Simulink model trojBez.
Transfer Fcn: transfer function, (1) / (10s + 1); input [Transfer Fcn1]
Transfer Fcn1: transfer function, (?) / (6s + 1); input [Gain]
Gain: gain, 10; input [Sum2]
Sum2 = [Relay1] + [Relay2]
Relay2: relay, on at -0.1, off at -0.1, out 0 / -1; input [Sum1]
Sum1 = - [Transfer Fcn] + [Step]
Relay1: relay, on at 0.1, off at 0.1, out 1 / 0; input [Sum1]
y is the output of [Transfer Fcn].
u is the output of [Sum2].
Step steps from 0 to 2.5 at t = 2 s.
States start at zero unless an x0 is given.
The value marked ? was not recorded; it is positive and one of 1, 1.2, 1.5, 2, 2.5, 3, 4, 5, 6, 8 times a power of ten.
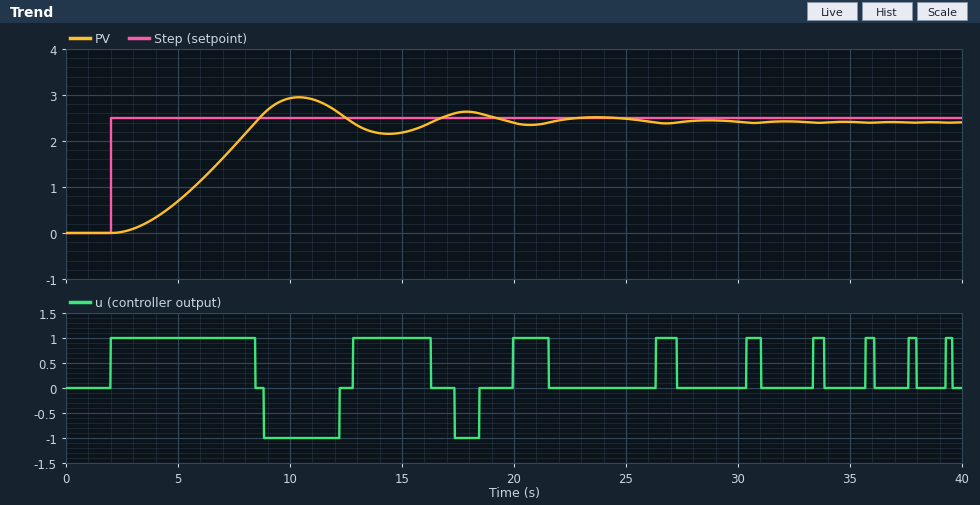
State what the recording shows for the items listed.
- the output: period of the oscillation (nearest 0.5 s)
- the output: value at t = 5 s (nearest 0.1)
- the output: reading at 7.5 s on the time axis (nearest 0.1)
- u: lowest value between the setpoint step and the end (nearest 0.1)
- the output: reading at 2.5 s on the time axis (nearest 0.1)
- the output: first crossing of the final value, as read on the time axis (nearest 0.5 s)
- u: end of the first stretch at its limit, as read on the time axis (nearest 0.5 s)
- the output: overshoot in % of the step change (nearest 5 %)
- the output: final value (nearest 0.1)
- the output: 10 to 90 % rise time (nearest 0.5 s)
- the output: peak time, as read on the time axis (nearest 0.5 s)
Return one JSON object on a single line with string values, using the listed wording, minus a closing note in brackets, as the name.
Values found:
{"the output: period of the oscillation": "7.5 s", "the output: value at t = 5 s": "0.7", "the output: reading at 7.5 s on the time axis": "1.9", "u: lowest value between the setpoint step and the end": "-1.0", "the output: reading at 2.5 s on the time axis": "0.0", "the output: first crossing of the final value, as read on the time axis": "8.5 s", "u: end of the first stretch at its limit, as read on the time axis": "8.5 s", "the output: overshoot in % of the step change": "25 %", "the output: final value": "2.4", "the output: 10 to 90 % rise time": "4.5 s", "the output: peak time, as read on the time axis": "10.5 s"}
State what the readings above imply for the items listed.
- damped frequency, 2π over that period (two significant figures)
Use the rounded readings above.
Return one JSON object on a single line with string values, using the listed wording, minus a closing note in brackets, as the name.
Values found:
{"damped frequency, 2π over that period": "0.84 rad/s"}
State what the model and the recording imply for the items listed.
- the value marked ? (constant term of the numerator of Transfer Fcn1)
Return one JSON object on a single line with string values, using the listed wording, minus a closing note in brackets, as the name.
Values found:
{"the value marked ?": "1.2"}
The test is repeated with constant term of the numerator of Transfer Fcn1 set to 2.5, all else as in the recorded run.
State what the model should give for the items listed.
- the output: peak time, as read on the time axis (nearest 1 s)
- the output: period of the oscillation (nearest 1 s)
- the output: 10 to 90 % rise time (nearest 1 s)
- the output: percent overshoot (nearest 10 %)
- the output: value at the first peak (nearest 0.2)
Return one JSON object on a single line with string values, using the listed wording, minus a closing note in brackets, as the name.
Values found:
{"the output: peak time, as read on the time axis": "8 s", "the output: period of the oscillation": "6 s", "the output: 10 to 90 % rise time": "3 s", "the output: percent overshoot": "40 %", "the output: value at the first peak": "3.2"}
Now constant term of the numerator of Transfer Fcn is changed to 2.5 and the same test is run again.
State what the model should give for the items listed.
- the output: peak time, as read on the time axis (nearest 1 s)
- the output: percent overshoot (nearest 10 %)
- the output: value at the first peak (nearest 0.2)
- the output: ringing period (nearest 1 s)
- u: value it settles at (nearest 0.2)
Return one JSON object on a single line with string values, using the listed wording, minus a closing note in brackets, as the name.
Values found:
{"the output: peak time, as read on the time axis": "7 s", "the output: percent overshoot": "40 %", "the output: value at the first peak": "3.4", "the output: ringing period": "6 s", "u: value it settles at": "0.0"}
